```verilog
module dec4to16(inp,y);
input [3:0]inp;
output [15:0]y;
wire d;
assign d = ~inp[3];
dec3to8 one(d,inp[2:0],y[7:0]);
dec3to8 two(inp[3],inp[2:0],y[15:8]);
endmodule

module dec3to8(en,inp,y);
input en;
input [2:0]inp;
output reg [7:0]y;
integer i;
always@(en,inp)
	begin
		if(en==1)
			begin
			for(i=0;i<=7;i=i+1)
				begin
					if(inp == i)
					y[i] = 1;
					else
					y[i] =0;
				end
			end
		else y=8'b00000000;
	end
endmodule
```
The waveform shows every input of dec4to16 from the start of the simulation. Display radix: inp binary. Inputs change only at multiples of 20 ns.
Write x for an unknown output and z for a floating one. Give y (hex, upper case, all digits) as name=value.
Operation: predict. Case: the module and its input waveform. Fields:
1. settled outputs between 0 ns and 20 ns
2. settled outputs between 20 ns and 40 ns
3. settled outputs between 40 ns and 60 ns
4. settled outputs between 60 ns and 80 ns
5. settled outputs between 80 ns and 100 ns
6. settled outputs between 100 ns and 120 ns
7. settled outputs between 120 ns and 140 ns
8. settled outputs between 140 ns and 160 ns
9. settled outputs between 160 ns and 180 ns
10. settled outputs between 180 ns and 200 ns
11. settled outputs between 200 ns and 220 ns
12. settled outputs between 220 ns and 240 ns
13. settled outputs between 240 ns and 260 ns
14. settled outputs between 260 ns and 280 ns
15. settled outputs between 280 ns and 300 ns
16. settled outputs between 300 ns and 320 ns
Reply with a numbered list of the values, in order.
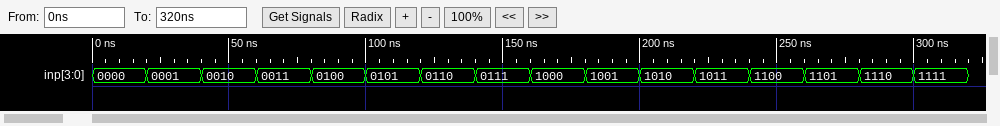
1. y=0001
2. y=0002
3. y=0004
4. y=0008
5. y=0010
6. y=0020
7. y=0040
8. y=0080
9. y=0100
10. y=0200
11. y=0400
12. y=0800
13. y=1000
14. y=2000
15. y=4000
16. y=8000
